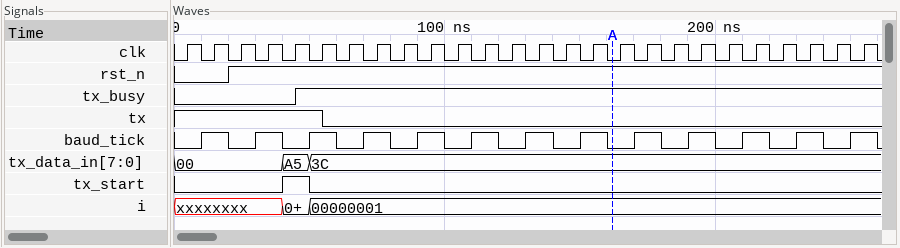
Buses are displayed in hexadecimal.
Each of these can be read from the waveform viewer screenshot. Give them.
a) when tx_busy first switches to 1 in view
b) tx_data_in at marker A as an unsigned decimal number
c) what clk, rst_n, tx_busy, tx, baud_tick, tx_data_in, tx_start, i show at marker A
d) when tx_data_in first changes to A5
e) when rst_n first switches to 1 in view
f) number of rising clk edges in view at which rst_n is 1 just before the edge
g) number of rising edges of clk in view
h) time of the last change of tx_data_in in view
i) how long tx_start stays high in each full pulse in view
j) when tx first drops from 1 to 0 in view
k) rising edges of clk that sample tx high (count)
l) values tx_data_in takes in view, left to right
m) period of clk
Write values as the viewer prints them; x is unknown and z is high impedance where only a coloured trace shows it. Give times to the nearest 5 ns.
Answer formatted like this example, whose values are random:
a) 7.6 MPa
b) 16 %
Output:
a) 45 ns
b) 60
c) clk=0, rst_n=1, tx_busy=1, tx=0, baud_tick=0, tx_data_in=3C, tx_start=0, i=00000001
d) 40 ns
e) 20 ns
f) 24
g) 26
h) 50 ns
i) 10 ns
j) 55 ns
k) 6
l) 00, A5, 3C
m) 10 ns
